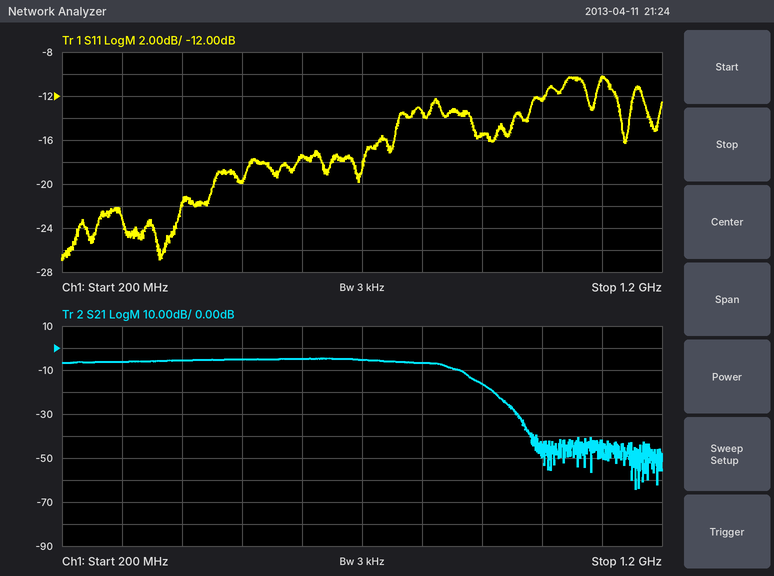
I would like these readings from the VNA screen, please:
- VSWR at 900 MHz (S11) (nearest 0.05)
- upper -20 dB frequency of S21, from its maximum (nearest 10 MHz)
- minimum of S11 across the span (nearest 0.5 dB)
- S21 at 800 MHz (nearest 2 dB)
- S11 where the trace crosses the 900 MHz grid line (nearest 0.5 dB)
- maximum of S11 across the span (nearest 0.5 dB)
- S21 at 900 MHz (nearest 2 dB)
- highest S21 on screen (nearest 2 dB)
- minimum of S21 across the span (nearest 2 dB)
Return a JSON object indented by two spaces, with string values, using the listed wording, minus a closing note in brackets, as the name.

{
  "VSWR at 900 MHz (S11)": "1.40",
  "upper -20 dB frequency of S21, from its maximum": "940 MHz",
  "minimum of S11 across the span": "-27.0 dB",
  "S21 at 800 MHz": "-6 dB",
  "S11 where the trace crosses the 900 MHz grid line": "-15.5 dB",
  "maximum of S11 across the span": "-10.0 dB",
  "S21 at 900 MHz": "-16 dB",
  "highest S21 on screen": "-4 dB",
  "minimum of S21 across the span": "-64 dB"
}
